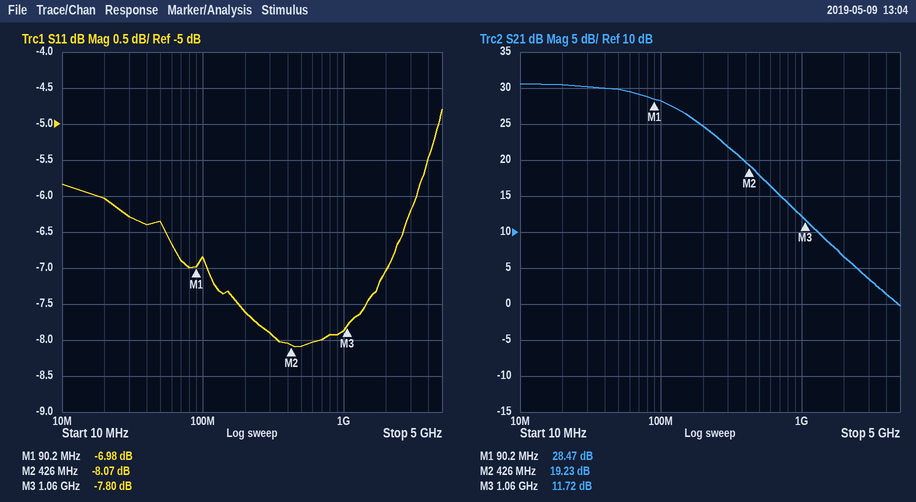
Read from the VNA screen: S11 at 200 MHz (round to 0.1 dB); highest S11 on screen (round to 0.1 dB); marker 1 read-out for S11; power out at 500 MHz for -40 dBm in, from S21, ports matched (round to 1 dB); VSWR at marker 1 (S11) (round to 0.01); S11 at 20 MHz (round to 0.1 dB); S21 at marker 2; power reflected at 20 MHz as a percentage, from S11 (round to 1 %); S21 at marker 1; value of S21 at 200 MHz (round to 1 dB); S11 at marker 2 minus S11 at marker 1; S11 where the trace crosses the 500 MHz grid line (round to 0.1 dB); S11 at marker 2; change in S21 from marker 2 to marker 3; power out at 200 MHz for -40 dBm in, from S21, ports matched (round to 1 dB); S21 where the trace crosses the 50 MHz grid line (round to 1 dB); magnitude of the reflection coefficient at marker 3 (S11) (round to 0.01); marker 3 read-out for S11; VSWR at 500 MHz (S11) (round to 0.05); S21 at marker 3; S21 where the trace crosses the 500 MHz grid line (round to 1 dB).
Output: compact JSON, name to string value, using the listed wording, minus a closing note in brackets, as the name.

{"S11 at 200 MHz": "-7.6 dB", "highest S11 on screen": "-4.8 dB", "marker 1 read-out for S11": "-6.98 dB", "power out at 500 MHz for -40 dBm in, from S21, ports matched": "-22 dBm", "VSWR at marker 1 (S11)": "2.62", "S11 at 20 MHz": "-6.0 dB", "S21 at marker 2": "19.23 dB", "power reflected at 20 MHz as a percentage, from S11": "25 %", "S21 at marker 1": "28.47 dB", "value of S21 at 200 MHz": "25 dB", "S11 at marker 2 minus S11 at marker 1": "-1.09 dB", "S11 where the trace crosses the 500 MHz grid line": "-8.1 dB", "S11 at marker 2": "-8.07 dB", "change in S21 from marker 2 to marker 3": "-7.51 dB", "power out at 200 MHz for -40 dBm in, from S21, ports matched": "-15 dBm", "S21 where the trace crosses the 50 MHz grid line": "30 dB", "magnitude of the reflection coefficient at marker 3 (S11)": "0.41", "marker 3 read-out for S11": "-7.80 dB", "VSWR at 500 MHz (S11)": "2.30", "S21 at marker 3": "11.72 dB", "S21 where the trace crosses the 500 MHz grid line": "18 dB"}
